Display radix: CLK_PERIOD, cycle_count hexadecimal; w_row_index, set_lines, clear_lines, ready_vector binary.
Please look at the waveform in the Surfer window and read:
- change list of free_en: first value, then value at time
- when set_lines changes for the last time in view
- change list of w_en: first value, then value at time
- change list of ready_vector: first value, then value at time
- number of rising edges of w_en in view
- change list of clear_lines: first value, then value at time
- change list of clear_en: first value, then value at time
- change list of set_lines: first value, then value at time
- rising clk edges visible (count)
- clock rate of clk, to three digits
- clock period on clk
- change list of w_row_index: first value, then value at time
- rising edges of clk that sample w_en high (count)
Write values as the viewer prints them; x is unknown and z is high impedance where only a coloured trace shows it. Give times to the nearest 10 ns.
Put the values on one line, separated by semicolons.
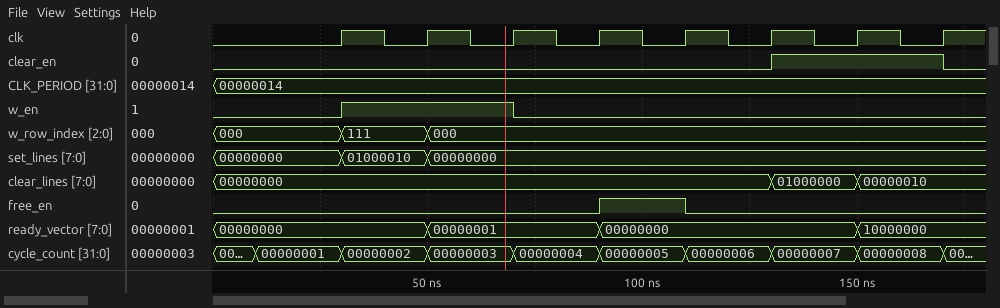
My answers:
0, 1 at 90 ns, 0 at 110 ns; 50 ns; 0, 1 at 30 ns, 0 at 70 ns; 00000000, 00000001 at 50 ns, 00000000 at 90 ns, 10000000 at 150 ns; 1; 00000000, 01000000 at 130 ns, 00000010 at 150 ns; 0, 1 at 130 ns, 0 at 170 ns; 00000000, 01000010 at 30 ns, 00000000 at 50 ns; 8; 50.0 MHz; 20 ns; 000, 111 at 30 ns, 000 at 50 ns; 2
